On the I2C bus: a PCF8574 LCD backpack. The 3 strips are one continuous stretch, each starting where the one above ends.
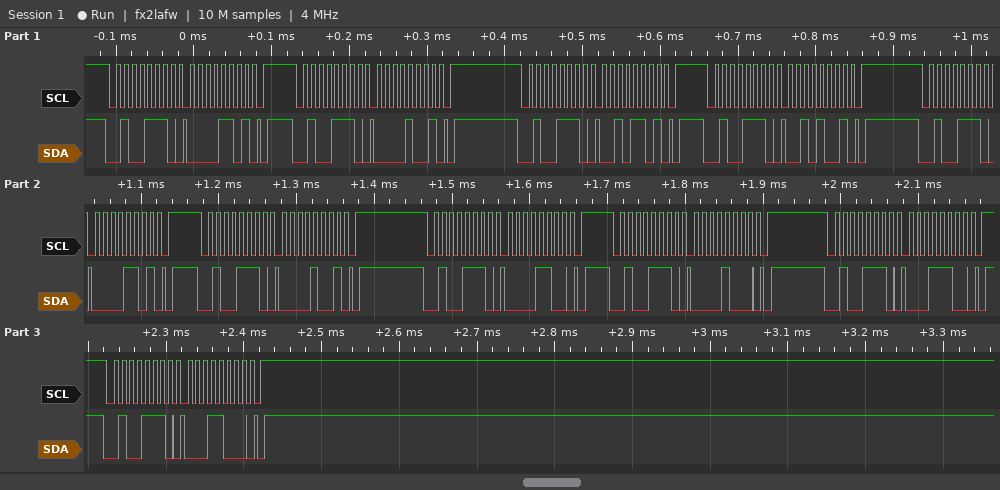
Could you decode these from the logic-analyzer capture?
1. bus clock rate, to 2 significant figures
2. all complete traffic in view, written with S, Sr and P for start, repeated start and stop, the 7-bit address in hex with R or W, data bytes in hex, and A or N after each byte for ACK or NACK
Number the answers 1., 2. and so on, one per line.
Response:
1. 100 kHz
2. S 27W A 0D A P S 27W A 09 A P S 27W A 2D A P S 27W A 29 A P S 27W A 0D A P S 27W A 09 A P S 27W A 0C A P S 27W A 08 A P S 27W A 1C A P S 27W A 18 A P
